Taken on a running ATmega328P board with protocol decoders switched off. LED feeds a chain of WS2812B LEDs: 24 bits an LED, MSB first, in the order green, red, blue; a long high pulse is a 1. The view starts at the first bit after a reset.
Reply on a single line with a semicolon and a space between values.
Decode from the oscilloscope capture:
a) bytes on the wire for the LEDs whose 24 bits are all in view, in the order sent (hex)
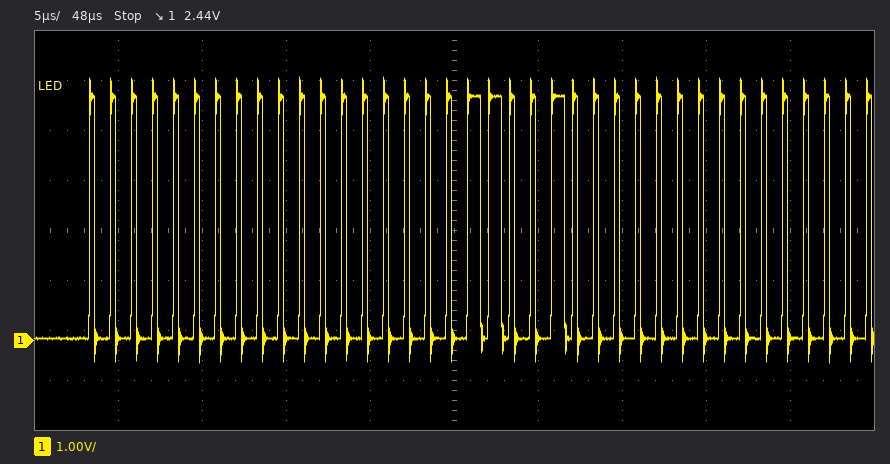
00 00 32
